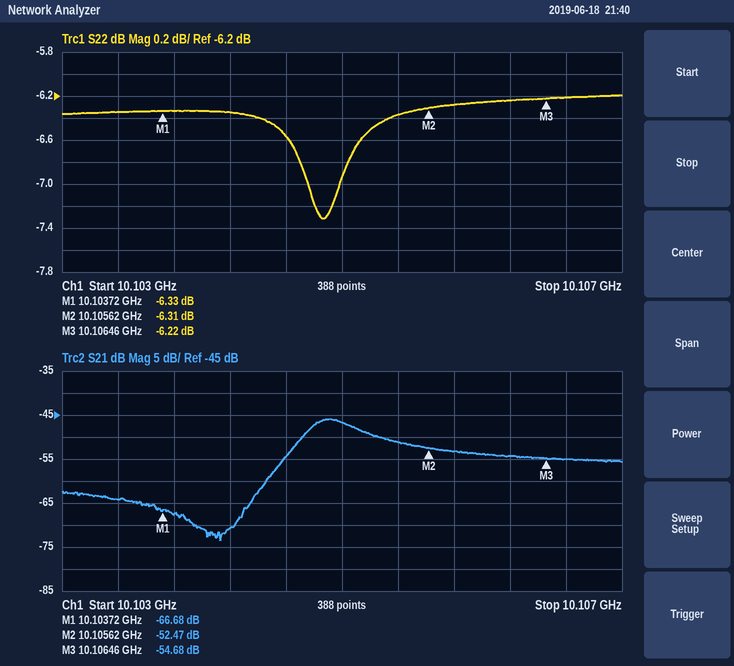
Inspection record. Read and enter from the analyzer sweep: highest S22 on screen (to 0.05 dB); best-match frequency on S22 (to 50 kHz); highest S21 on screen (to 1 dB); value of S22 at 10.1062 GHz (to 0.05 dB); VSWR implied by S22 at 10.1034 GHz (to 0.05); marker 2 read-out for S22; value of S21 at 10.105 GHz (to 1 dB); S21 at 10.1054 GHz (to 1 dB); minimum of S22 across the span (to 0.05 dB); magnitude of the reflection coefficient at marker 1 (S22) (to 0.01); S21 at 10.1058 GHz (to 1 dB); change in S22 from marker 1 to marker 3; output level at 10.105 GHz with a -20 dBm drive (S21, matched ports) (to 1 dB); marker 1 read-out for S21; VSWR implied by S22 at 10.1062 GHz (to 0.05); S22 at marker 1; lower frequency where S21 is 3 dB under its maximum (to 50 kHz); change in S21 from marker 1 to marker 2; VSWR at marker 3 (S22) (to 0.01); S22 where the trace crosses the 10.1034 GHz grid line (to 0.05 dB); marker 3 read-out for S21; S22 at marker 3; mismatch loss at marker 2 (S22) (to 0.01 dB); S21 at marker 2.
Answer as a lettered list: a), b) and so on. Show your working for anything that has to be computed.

a) -6.20 dB
b) 10.10485 GHz
c) -46 dB
d) -6.25 dB
e) |Γ| = 10^(-6.35/20) = 0.4814; VSWR = (1 + 0.4814)/(1 − 0.4814) ≈ 2.86, so 2.85 to the nearest 0.05
f) -6.31 dB
g) -47 dB
h) -51 dB
i) -7.30 dB
j) 10^(-6.33/20) ≈ 0.48
k) -53 dB
l) -6.22 − (-6.33) = 0.11 dB
m) -20 dBm + (-47 dB) = -67 dBm
n) -66.68 dB
o) |Γ| = 10^(-6.25/20) = 0.4870; VSWR = (1 + 0.4870)/(1 − 0.4870) ≈ 2.90
p) -6.33 dB
q) 10.10475 GHz
r) -52.47 − (-66.68) = 14.21 dB
s) (1 + 0.4887)/(1 − 0.4887) ≈ 2.91
t) -6.35 dB
u) -54.68 dB
v) -6.22 dB
w) −10 log10(1 − 10^(-6.31/10)) ≈ 1.16 dB
x) -52.47 dB
